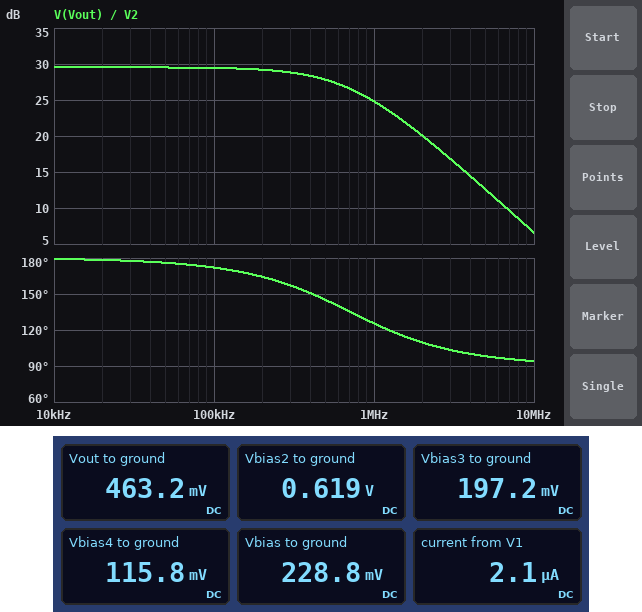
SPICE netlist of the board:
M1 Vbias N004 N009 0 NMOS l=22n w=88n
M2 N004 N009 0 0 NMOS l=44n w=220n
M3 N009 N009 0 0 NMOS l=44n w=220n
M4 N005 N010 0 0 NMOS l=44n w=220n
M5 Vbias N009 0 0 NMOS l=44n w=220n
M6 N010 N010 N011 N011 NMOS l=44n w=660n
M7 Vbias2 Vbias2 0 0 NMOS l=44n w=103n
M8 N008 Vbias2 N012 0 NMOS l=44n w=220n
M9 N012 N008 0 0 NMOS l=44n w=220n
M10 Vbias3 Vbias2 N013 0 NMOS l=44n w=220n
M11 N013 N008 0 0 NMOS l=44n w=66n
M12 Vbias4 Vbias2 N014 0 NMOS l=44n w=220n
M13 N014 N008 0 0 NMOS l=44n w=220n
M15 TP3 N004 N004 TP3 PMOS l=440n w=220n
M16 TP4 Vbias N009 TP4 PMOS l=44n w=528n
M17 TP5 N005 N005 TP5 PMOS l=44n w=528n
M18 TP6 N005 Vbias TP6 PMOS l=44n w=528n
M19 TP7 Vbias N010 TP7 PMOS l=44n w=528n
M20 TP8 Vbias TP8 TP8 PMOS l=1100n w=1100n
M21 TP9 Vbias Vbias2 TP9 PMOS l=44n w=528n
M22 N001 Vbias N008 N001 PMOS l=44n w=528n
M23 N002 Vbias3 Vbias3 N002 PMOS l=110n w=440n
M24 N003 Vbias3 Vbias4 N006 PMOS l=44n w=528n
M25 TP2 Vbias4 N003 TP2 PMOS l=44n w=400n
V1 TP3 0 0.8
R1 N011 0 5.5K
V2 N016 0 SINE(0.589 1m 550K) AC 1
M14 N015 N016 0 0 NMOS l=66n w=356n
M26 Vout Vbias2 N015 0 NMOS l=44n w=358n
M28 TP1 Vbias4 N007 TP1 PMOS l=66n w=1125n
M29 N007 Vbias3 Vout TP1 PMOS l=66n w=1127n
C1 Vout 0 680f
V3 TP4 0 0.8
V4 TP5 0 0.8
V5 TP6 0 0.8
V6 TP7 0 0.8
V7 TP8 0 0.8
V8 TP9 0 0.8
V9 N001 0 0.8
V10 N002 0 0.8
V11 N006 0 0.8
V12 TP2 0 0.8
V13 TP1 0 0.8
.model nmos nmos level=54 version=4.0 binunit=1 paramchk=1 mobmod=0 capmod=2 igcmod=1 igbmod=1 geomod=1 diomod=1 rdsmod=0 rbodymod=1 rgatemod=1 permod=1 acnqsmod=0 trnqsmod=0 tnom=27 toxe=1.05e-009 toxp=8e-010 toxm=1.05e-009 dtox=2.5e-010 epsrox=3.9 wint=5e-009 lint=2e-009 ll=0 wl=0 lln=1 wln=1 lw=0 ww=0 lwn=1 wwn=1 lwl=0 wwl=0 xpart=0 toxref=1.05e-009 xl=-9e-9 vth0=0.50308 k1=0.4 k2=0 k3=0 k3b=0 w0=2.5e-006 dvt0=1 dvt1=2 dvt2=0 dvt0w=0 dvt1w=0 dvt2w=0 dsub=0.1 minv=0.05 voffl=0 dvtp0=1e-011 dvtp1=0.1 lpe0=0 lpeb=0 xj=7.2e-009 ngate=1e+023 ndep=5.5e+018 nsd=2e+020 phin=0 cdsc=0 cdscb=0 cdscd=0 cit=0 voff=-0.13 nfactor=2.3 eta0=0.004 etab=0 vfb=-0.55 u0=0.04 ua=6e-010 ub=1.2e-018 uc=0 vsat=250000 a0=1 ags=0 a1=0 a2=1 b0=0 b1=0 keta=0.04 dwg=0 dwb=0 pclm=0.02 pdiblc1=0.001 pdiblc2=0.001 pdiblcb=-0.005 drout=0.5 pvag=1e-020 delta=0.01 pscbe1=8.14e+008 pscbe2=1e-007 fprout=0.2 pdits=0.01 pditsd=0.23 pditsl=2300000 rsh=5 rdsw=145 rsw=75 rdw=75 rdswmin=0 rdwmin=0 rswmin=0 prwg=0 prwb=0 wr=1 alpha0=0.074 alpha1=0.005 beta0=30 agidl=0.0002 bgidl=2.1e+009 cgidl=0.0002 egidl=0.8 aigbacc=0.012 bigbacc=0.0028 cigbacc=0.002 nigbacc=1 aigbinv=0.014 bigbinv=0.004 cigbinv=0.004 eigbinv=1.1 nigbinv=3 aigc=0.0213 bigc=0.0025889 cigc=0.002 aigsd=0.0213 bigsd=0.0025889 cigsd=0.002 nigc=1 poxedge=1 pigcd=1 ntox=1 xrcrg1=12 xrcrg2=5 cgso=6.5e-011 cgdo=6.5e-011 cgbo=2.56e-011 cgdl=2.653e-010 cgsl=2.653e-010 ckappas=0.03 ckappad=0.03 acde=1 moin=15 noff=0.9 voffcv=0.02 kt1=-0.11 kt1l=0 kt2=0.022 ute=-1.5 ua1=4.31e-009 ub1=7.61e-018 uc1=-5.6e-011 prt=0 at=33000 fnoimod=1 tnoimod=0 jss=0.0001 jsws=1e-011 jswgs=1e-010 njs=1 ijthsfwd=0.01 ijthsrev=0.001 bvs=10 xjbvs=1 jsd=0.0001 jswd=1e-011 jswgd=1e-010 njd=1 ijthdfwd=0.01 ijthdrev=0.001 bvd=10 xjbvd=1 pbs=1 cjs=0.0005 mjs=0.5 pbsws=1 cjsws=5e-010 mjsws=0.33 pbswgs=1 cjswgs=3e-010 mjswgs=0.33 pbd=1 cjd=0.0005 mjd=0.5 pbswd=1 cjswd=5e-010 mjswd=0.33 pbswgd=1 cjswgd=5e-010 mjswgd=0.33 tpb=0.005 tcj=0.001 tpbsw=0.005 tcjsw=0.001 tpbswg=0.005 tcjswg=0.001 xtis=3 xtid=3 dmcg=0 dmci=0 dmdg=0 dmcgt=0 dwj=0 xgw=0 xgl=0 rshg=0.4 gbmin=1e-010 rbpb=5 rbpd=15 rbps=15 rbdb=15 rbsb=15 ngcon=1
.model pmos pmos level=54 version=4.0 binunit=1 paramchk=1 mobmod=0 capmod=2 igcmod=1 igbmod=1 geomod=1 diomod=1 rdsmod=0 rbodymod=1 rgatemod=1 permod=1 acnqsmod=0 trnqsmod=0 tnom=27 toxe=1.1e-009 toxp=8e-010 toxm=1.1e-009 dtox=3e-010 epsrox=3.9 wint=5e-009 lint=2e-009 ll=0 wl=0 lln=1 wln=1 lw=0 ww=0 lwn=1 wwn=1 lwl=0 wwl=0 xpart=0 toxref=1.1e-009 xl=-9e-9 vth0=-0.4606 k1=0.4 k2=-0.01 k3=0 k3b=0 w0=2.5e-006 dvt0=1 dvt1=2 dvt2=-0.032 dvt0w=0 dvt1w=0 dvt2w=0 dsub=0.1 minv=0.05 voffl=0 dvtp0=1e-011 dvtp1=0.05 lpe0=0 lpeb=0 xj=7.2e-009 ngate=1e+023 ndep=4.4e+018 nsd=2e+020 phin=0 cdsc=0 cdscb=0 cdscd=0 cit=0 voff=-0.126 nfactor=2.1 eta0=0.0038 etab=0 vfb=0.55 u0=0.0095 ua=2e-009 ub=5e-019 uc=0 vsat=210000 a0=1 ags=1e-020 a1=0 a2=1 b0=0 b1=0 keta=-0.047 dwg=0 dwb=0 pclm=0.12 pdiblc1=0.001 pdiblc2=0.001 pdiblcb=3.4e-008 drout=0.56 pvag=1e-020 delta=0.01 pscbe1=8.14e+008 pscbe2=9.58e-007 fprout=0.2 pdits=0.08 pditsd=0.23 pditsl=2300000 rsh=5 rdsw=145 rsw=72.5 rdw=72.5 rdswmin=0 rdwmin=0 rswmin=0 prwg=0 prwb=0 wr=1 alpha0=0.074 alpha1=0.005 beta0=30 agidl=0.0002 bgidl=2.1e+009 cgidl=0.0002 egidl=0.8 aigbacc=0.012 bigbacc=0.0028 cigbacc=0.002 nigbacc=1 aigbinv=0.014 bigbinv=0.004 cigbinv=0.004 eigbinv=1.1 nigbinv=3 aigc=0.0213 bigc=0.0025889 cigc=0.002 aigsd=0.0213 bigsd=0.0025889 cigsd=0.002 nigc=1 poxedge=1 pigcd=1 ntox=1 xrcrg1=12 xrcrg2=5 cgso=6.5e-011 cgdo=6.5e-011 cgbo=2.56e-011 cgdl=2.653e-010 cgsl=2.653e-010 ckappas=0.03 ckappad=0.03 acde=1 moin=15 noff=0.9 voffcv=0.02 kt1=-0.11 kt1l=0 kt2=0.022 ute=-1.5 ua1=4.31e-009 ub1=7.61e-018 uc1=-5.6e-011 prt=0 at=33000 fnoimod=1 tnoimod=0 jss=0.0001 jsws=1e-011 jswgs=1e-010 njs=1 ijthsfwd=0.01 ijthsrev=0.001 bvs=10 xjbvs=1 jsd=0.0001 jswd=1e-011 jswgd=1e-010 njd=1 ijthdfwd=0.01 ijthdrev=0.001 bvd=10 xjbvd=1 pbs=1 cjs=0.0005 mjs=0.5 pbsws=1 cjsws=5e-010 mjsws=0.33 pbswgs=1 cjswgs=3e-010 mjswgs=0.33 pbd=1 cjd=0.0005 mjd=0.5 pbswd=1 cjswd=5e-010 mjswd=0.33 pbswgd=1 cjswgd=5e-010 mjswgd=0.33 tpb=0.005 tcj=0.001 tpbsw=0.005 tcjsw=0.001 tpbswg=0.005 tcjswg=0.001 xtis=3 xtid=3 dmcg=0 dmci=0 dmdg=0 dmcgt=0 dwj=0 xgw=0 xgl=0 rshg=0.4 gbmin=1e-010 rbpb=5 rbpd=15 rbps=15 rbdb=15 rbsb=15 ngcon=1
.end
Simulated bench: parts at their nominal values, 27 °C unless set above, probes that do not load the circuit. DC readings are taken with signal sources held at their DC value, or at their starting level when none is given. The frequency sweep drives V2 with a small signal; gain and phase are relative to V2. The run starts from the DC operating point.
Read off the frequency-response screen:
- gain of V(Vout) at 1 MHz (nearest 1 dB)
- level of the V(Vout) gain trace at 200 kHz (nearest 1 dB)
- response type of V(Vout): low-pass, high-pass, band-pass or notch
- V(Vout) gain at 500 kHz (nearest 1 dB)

25 dB
29 dB
low-pass
28 dB
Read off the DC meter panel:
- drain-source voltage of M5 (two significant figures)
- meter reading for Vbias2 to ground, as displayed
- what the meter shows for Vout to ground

230 mV
0.619 V
463.2 mV
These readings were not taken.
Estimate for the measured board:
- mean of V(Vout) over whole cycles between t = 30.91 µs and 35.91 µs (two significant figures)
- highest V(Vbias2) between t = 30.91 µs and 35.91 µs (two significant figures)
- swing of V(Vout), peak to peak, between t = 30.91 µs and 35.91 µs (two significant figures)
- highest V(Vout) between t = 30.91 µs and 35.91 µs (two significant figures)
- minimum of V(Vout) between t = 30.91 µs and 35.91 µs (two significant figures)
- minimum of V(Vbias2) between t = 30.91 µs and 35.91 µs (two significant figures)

460 mV
620 mV
47 mV
490 mV
440 mV
620 mV
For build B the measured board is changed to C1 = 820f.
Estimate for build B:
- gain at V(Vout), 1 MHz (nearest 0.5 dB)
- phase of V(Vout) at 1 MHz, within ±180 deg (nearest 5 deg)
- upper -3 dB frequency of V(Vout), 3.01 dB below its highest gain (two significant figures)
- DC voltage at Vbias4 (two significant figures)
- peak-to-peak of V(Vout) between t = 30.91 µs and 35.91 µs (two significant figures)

23.5 dB
120 deg
590 kHz
120 mV
44 mV
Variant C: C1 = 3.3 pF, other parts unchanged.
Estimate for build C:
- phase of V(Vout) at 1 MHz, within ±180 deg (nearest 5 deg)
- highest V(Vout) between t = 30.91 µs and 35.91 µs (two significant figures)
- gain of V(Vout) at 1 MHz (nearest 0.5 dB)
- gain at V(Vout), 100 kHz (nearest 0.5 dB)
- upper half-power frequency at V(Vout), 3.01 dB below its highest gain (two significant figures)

100 deg
470 mV
13.0 dB
28.0 dB
150 kHz
